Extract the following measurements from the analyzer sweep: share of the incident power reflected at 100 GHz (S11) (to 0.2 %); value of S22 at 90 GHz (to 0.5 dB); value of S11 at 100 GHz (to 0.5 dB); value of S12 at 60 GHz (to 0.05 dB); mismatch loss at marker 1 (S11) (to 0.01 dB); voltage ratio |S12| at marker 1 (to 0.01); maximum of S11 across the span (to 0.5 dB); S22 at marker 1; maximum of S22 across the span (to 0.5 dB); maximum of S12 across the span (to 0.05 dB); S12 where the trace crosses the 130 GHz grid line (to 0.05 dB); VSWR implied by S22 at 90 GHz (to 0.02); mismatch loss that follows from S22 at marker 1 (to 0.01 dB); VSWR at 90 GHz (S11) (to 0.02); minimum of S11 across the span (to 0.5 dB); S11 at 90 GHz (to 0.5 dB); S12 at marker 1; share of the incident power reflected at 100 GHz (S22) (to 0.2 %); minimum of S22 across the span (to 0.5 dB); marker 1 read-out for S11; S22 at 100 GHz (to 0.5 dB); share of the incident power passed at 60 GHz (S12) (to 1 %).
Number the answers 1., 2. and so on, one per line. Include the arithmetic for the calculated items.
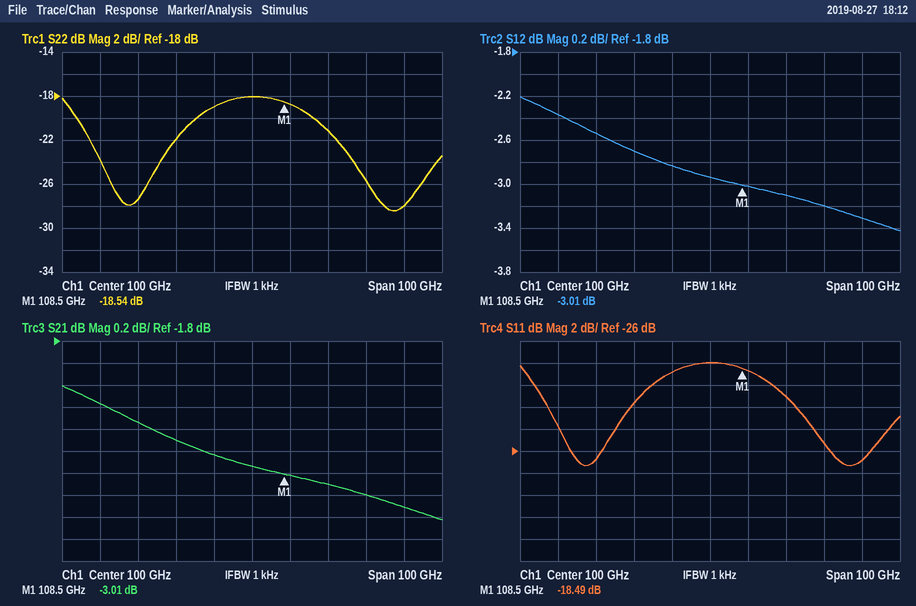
1. 10^(-18/10) ≈ 1.6 %
2. -19.0 dB
3. -18.0 dB
4. -2.35 dB
5. −10 log10(1 − 10^(-18.49/10)) ≈ 0.06 dB
6. 10^(-3.01/20) ≈ 0.71
7. -18.0 dB
8. -18.54 dB
9. -18.0 dB
10. -2.20 dB
11. -3.20 dB
12. |Γ| = 10^(-19/20) = 0.1122; VSWR = (1 + 0.1122)/(1 − 0.1122) ≈ 1.25, so 1.26 to the nearest 0.02
13. −10 log10(1 − 10^(-18.54/10)) ≈ 0.06 dB
14. |Γ| = 10^(-19/20) = 0.1122; VSWR = (1 + 0.1122)/(1 − 0.1122) ≈ 1.25, so 1.26 to the nearest 0.02
15. -27.5 dB
16. -19.0 dB
17. -3.01 dB
18. 10^(-18/10) ≈ 1.6 %
19. -28.5 dB
20. -18.49 dB
21. -18.0 dB
22. 10^(-2.35/10) ≈ 58 %
